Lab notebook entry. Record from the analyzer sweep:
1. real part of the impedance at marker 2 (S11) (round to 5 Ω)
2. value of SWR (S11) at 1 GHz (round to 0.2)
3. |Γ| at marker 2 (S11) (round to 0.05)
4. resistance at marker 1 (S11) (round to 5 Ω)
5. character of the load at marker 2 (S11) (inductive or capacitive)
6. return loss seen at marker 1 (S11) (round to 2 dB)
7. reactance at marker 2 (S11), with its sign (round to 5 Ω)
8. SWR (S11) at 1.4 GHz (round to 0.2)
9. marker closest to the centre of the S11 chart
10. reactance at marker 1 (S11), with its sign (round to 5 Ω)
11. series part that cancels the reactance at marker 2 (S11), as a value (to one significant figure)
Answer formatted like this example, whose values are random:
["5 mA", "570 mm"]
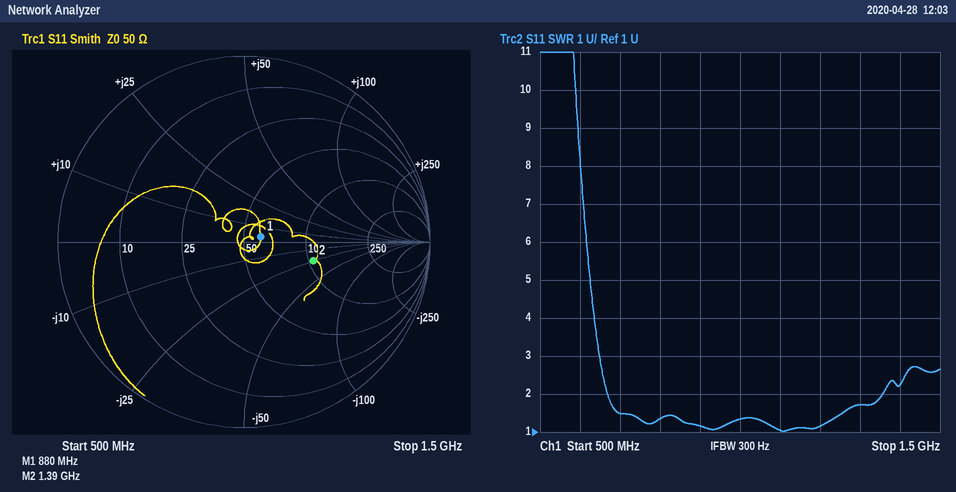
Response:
["105 Ω", "1.4", "0.40", "60 Ω", "capacitive", "20 dB", "-25 Ω", "2.2", "marker 1", "+5 Ω", "3 nH"]
